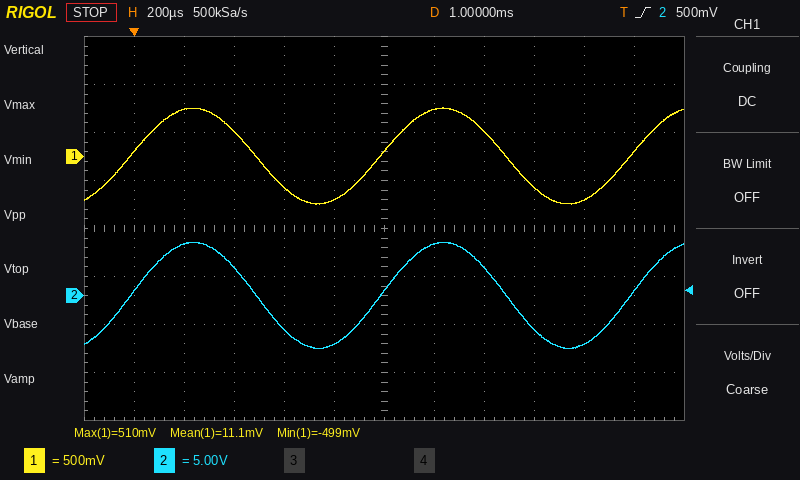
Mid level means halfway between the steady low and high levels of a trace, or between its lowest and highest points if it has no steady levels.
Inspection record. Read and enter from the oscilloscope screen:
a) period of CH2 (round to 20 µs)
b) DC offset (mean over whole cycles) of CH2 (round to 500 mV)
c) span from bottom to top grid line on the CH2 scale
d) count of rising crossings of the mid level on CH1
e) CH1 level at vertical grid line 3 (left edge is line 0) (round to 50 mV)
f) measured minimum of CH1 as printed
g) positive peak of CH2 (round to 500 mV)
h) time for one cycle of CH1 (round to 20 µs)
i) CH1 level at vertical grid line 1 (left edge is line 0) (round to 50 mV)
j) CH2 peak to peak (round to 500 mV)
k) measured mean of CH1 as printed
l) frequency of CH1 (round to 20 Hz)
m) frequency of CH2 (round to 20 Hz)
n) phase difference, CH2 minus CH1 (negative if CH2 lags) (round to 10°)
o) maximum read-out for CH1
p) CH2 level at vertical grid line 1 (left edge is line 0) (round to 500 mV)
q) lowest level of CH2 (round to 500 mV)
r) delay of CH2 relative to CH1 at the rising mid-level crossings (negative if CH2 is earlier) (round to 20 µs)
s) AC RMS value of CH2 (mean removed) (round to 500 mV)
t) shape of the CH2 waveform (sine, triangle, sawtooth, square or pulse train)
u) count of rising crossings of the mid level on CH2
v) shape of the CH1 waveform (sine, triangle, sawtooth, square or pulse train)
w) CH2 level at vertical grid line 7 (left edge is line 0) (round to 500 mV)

1.00 ms
0.0 V
40 V
3
250 mV
-499 mV
5.5 V
1.00 ms
50 mV
11.0 V
11.1 mV
1.00 kHz
1.00 kHz
0°
510 mV
500 mV
-5.5 V
0 µs
4.0 V
sine
3
sine
5.5 V
